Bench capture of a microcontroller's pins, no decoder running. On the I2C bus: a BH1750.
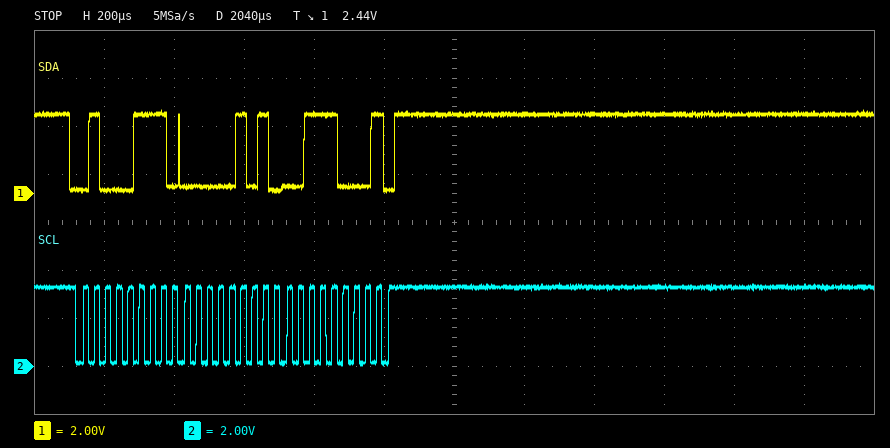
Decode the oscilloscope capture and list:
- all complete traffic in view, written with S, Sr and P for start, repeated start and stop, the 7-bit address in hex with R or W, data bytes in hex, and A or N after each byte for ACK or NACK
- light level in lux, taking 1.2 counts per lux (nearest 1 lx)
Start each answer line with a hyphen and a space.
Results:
- S 23R A 05 A 38 N P
- 1113 lx
